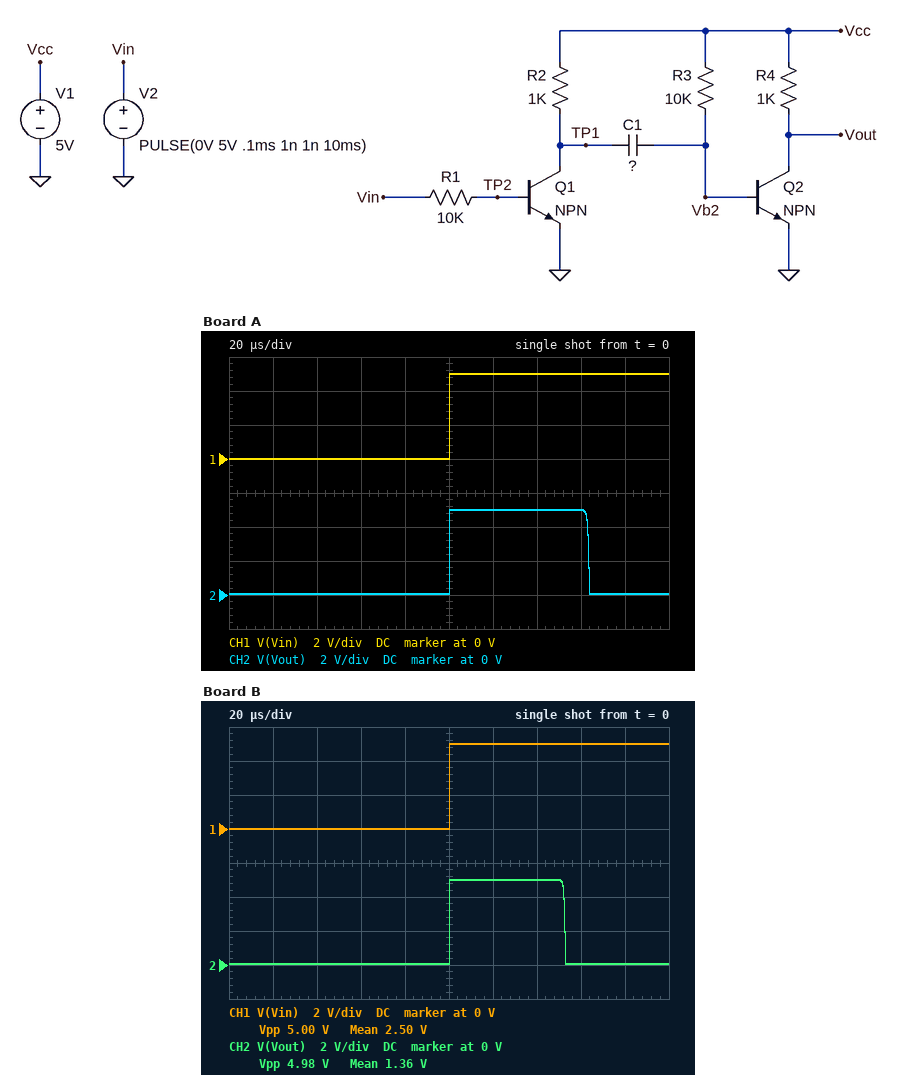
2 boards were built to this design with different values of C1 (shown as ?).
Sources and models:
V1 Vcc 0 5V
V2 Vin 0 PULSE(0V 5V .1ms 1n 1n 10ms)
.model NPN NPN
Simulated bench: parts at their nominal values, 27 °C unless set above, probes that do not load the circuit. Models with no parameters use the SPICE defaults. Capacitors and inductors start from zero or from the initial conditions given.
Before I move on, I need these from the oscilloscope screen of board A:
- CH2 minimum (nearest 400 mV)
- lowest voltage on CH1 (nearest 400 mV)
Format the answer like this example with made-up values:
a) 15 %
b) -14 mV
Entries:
a) 0 V
b) 0 V
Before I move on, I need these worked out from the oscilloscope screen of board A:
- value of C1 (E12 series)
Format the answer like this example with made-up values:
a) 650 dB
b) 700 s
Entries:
a) 8.2 nF
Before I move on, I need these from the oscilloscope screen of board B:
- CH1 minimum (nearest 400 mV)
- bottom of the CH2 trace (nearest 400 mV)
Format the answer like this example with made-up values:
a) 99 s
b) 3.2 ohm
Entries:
a) 0 V
b) 0 V
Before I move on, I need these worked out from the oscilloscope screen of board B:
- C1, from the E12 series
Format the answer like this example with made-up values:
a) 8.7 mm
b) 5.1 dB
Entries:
a) 6.8 nF
